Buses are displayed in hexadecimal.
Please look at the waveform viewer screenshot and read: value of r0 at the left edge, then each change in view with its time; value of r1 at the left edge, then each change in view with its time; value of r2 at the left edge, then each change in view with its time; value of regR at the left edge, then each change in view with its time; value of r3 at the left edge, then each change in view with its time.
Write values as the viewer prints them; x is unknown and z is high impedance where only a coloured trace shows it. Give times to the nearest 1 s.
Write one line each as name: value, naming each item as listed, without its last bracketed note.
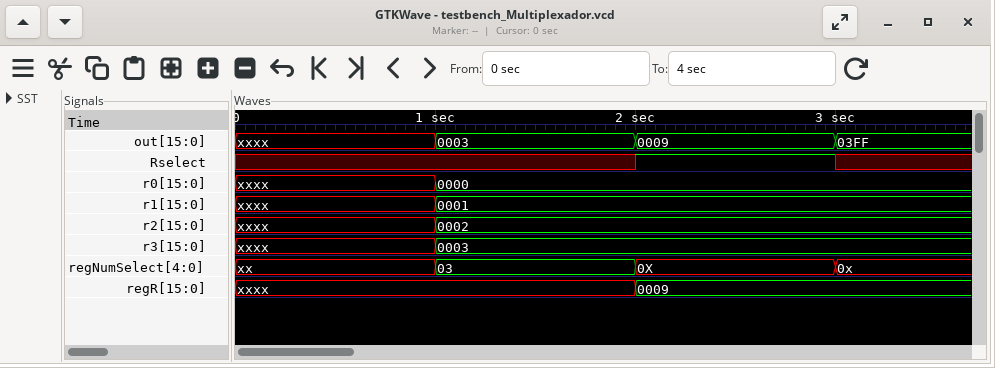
value of r0 at the left edge, then each change in view with its time: xxxx, 0000 at 1 s
value of r1 at the left edge, then each change in view with its time: xxxx, 0001 at 1 s
value of r2 at the left edge, then each change in view with its time: xxxx, 0002 at 1 s
value of regR at the left edge, then each change in view with its time: xxxx, 0009 at 2 s
value of r3 at the left edge, then each change in view with its time: xxxx, 0003 at 1 s
